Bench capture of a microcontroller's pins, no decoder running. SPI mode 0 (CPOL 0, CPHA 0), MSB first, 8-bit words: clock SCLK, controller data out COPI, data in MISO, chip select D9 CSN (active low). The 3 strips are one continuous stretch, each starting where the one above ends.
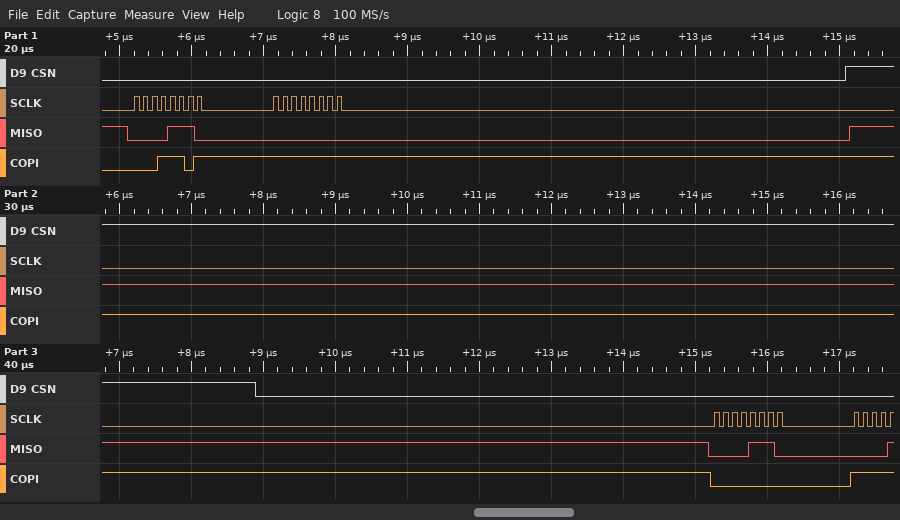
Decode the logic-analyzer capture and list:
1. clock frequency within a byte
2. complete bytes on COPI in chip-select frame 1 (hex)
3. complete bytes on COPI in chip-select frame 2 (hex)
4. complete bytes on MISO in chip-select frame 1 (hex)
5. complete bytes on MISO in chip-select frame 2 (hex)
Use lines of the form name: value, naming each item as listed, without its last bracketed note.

clock frequency within a byte: 8 MHz
complete bytes on COPI in chip-select frame 1: 1D FF
complete bytes on COPI in chip-select frame 2: 00
complete bytes on MISO in chip-select frame 1: 0E 00
complete bytes on MISO in chip-select frame 2: 0E
